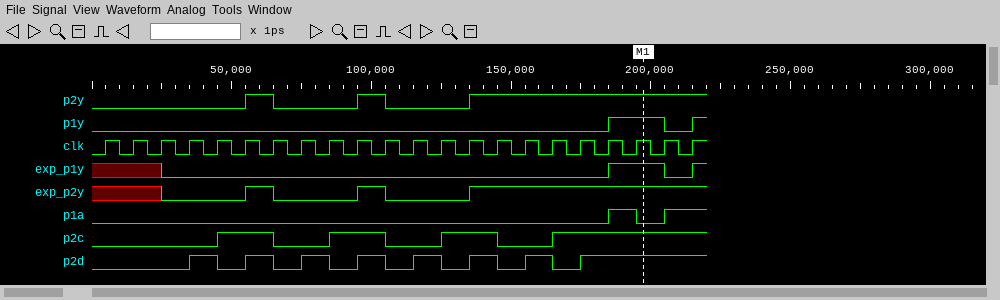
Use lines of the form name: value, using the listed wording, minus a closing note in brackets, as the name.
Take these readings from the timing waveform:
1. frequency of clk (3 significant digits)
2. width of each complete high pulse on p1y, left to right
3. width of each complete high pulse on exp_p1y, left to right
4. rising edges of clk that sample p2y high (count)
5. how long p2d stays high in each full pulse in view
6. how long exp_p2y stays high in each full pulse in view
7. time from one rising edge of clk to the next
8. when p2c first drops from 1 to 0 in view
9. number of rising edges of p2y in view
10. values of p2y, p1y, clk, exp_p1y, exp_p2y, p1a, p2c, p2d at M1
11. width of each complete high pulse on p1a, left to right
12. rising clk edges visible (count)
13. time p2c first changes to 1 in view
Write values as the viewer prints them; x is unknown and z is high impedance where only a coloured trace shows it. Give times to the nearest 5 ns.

frequency of clk: 100 MHz
width of each complete high pulse on p1y, left to right: 20 ns
width of each complete high pulse on exp_p1y, left to right: 20 ns
rising edges of clk that sample p2y high: 10
how long p2d stays high in each full pulse in view: 10 ns, 10 ns, 10 ns, 10 ns, 10 ns, 10 ns, 10 ns
how long exp_p2y stays high in each full pulse in view: 10 ns, 10 ns
time from one rising edge of clk to the next: 10 ns
when p2c first drops from 1 to 0 in view: 65 ns
number of rising edges of p2y in view: 3
values of p2y, p1y, clk, exp_p1y, exp_p2y, p1a, p2c, p2d at M1: p2y=1, p1y=1, clk=1, exp_p1y=1, exp_p2y=1, p1a=0, p2c=1, p2d=1
width of each complete high pulse on p1a, left to right: 10 ns
rising clk edges visible: 22
time p2c first changes to 1 in view: 45 ns
